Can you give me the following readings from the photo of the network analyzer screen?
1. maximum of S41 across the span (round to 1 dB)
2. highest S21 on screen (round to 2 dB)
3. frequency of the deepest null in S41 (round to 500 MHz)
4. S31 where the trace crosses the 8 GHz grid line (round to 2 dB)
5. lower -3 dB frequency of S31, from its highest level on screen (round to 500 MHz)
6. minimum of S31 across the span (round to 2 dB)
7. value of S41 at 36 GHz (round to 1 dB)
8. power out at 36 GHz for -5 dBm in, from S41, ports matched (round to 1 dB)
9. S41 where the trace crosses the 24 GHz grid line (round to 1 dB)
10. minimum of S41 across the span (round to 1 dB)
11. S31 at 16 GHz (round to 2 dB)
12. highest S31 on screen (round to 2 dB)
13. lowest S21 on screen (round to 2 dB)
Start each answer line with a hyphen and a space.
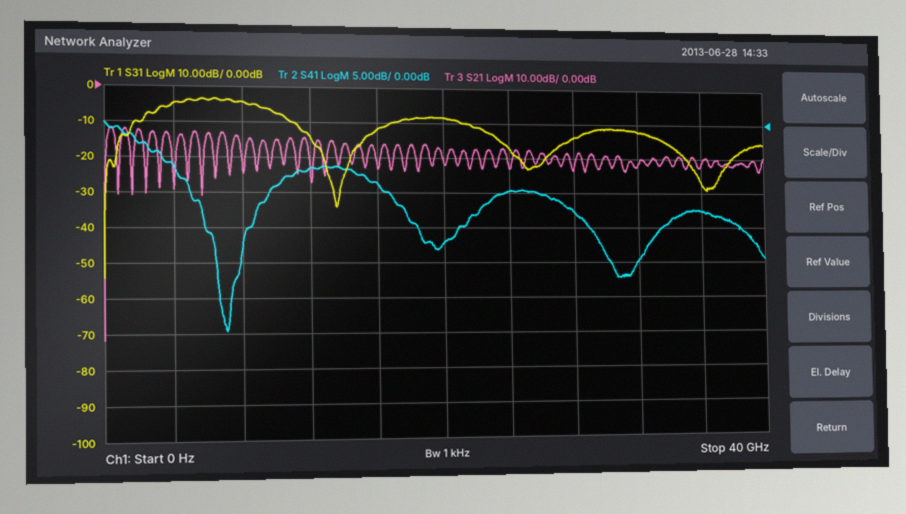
- 0 dB
- -12 dB
- 7.0 GHz
- -4 dB
- 3.0 GHz
- -54 dB
- -13 dB
- -18 dBm
- -10 dB
- -30 dB
- -12 dB
- -4 dB
- -72 dB
